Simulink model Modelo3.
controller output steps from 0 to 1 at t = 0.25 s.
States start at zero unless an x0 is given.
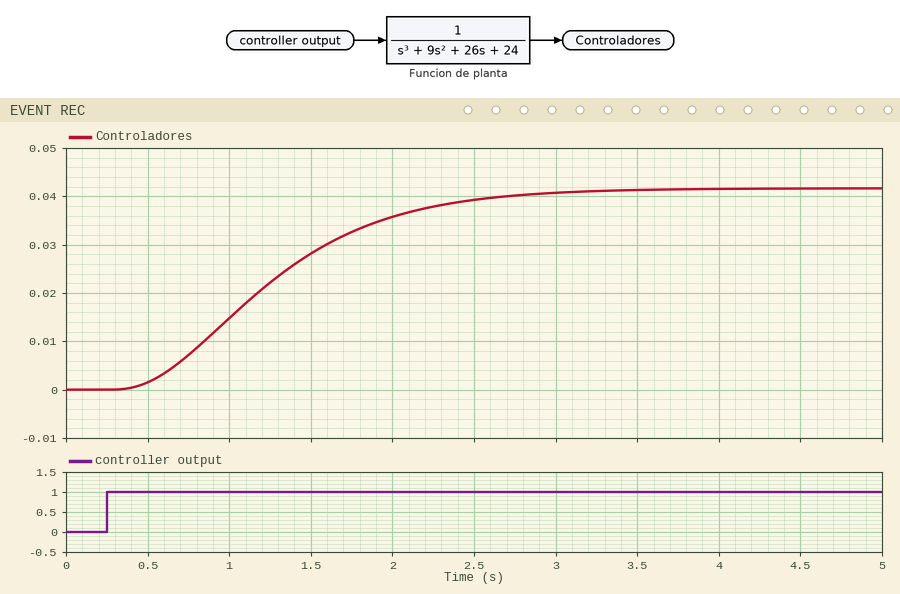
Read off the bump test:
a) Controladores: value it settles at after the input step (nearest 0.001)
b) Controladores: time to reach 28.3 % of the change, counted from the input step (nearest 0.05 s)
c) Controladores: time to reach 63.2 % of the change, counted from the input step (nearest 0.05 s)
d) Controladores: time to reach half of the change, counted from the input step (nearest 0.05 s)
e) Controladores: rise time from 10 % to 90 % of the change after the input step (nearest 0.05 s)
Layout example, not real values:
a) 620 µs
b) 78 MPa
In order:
a) 0.042
b) 0.65 s
c) 1.15 s
d) 0.95 s
e) 1.55 s
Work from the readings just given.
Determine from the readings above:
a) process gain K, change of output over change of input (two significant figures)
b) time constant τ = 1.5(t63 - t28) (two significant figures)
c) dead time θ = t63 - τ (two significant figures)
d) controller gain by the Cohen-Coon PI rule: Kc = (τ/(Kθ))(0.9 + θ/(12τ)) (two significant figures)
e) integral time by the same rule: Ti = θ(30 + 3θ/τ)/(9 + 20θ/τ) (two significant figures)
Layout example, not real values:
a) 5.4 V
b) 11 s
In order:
a) 0.042
b) 0.75 s
c) 0.40 s
d) 42
e) 0.64 s
